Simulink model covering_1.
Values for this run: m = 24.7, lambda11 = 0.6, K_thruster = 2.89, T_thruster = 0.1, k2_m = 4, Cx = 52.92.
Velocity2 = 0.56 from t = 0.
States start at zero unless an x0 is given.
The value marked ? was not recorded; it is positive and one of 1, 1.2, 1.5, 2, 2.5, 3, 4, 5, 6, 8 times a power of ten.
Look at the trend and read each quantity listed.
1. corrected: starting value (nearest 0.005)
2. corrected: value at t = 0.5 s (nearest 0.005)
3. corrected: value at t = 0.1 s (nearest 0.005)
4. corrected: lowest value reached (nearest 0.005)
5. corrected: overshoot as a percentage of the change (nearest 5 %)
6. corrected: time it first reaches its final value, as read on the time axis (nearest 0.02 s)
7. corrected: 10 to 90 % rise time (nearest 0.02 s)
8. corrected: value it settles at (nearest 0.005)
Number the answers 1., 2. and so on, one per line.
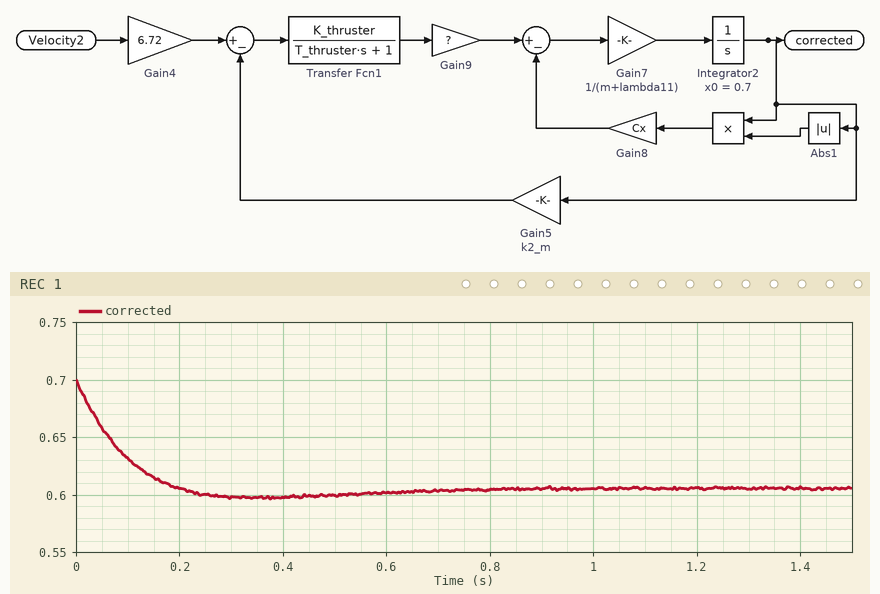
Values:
1. 0.700
2. 0.600
3. 0.630
4. 0.595
5. 10 %
6. 0.20 s
7. 0.14 s
8. 0.605
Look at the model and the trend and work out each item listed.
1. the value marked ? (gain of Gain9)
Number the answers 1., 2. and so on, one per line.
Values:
1. 5
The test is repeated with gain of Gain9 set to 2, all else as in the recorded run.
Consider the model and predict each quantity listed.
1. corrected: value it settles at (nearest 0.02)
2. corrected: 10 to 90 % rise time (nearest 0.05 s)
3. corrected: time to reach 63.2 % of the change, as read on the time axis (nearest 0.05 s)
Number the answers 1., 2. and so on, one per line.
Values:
1. 0.46
2. 0.60 s
3. 0.25 s
